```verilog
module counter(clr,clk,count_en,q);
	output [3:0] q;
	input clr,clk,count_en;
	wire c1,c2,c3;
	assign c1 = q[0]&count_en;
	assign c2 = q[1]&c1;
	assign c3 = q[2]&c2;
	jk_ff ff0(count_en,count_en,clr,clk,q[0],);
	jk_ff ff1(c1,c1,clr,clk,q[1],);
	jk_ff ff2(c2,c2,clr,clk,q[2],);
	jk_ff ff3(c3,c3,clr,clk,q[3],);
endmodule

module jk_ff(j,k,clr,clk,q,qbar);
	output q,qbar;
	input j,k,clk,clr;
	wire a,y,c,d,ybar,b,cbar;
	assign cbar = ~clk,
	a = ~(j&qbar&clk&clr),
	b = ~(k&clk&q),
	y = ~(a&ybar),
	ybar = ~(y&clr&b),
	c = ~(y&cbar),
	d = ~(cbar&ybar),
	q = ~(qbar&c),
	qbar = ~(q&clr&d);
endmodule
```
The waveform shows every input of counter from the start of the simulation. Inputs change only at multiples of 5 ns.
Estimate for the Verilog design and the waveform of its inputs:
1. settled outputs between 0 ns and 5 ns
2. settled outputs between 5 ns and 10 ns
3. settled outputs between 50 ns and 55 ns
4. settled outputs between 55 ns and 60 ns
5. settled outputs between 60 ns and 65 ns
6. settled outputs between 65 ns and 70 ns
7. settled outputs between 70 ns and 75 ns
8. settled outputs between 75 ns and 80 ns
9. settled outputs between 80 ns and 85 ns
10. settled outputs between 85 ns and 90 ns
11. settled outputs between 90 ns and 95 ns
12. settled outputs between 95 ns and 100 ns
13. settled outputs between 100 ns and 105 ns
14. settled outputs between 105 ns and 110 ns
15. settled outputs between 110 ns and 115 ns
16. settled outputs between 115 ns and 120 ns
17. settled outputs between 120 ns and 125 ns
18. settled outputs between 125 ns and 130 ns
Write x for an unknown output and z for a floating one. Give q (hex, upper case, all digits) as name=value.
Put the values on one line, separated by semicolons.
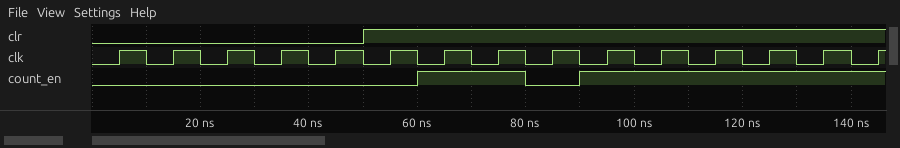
q=0; q=0; q=0; q=0; q=0; q=0; q=1; q=1; q=2; q=2; q=2; q=2; q=3; q=3; q=4; q=4; q=5; q=5
